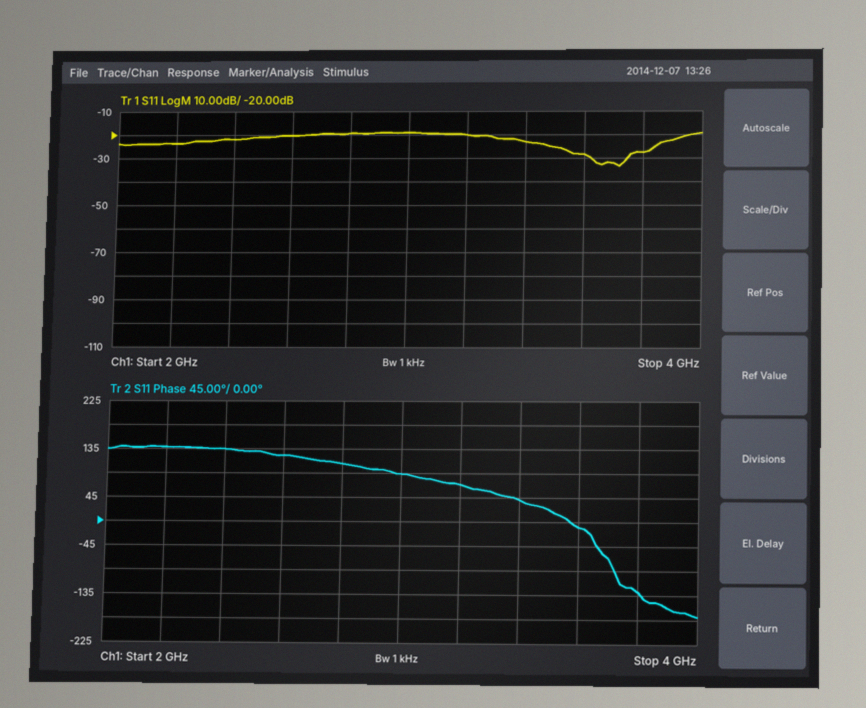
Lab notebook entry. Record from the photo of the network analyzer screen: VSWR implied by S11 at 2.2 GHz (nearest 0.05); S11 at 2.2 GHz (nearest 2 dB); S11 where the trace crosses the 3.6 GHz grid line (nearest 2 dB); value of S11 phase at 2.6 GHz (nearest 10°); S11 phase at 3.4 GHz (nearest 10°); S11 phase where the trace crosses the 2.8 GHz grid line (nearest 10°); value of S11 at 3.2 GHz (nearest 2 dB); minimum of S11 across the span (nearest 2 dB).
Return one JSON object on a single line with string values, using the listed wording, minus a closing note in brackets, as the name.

{"VSWR implied by S11 at 2.2 GHz": "1.15", "S11 at 2.2 GHz": "-24 dB", "S11 where the trace crosses the 3.6 GHz grid line": "-28 dB", "value of S11 phase at 2.6 GHz": "120°", "S11 phase at 3.4 GHz": "40°", "S11 phase where the trace crosses the 2.8 GHz grid line": "110°", "value of S11 at 3.2 GHz": "-20 dB", "minimum of S11 across the span": "-34 dB"}
